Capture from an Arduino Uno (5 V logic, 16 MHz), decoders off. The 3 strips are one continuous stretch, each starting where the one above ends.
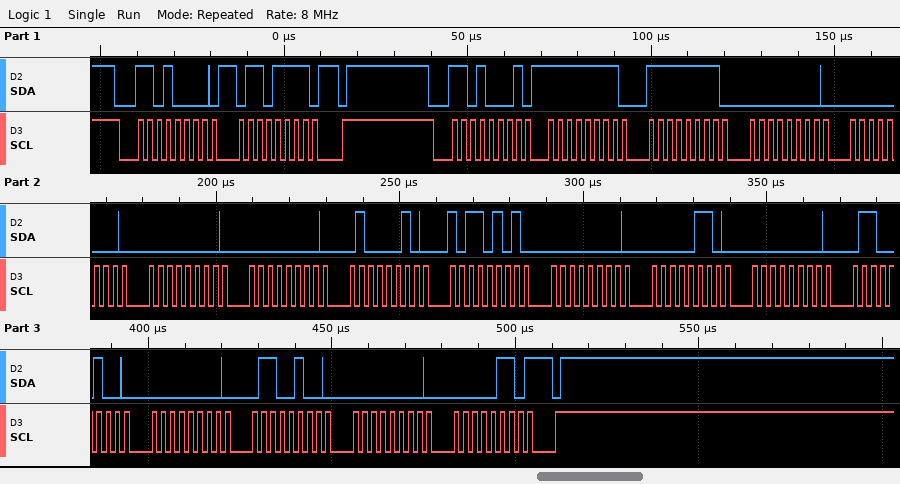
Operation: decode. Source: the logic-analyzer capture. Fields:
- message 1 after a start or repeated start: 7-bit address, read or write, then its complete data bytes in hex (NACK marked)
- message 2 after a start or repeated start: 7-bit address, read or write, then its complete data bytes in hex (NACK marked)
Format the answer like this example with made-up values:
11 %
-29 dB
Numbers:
0x68 write: 6F
0x68 read: FF FF 00 00 00 00 42 B5 00 06 00 64 00 64 00 06 NACK
